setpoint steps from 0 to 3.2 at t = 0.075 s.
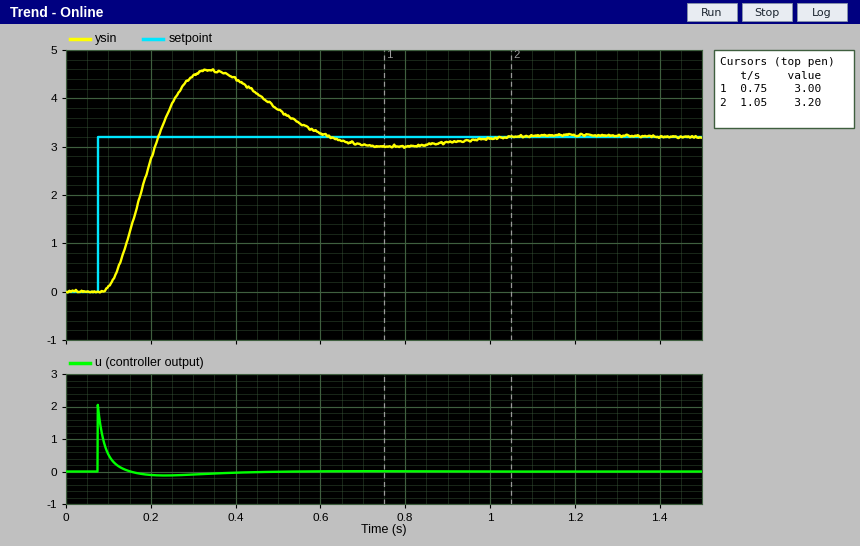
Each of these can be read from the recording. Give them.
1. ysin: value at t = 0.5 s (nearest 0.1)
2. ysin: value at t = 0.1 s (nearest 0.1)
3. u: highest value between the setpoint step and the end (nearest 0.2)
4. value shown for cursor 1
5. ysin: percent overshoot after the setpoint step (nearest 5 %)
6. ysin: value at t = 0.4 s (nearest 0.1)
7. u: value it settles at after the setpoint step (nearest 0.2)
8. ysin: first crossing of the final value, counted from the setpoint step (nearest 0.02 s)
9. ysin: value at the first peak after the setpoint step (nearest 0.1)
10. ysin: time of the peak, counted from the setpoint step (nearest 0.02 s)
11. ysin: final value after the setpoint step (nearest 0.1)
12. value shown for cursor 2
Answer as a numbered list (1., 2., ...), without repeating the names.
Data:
1. 3.8
2. 0.1
3. 2.0
4. 3.00
5. 45 %
6. 4.4
7. 0.0
8. 0.14 s
9. 4.6
10. 0.26 s
11. 3.2
12. 3.20
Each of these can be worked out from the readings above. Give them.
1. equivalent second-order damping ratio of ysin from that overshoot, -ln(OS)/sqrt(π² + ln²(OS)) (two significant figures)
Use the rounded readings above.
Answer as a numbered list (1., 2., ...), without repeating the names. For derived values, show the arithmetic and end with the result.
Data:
1. ln(0.45) = -0.799; 0.799 / sqrt(9.870 + 0.638) = 0.25
